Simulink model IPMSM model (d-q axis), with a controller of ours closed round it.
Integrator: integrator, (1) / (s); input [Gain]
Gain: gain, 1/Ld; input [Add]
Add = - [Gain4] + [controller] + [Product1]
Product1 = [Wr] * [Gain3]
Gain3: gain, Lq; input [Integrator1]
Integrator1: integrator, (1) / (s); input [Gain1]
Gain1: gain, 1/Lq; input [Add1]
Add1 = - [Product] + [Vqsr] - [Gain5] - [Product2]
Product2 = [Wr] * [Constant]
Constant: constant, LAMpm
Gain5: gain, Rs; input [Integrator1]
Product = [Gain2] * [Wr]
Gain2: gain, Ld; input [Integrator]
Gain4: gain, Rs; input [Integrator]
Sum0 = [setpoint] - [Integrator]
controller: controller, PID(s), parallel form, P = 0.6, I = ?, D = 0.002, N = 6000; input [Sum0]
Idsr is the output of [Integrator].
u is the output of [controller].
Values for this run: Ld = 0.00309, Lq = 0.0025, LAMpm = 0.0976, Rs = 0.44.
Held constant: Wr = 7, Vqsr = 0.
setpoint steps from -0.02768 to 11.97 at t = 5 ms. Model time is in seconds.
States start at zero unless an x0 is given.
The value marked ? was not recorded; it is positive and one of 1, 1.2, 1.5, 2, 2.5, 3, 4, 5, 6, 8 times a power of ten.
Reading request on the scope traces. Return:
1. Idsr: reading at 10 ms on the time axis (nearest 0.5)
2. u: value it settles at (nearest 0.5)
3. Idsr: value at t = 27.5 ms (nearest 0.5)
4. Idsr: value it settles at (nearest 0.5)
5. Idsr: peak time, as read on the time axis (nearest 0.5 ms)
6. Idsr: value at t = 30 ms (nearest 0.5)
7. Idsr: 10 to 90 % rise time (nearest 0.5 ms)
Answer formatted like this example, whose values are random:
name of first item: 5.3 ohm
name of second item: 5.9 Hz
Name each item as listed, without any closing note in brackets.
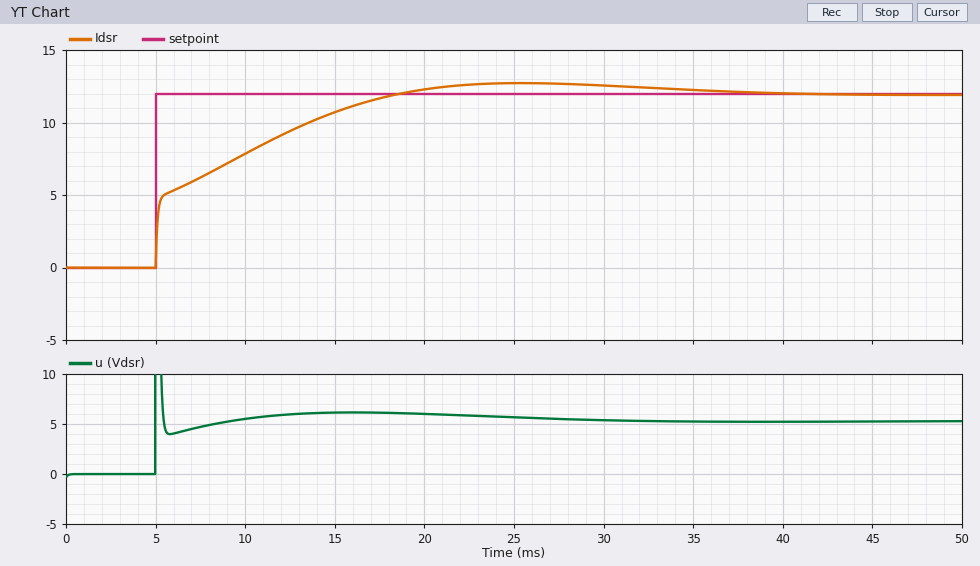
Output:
Idsr: reading at 10 ms on the time axis: 8.0
u: value it settles at: 5.5
Idsr: value at t = 27.5 ms: 12.5
Idsr: value it settles at: 12.0
Idsr: peak time, as read on the time axis: 25.5 ms
Idsr: value at t = 30 ms: 12.5
Idsr: 10 to 90 % rise time: 10.0 ms
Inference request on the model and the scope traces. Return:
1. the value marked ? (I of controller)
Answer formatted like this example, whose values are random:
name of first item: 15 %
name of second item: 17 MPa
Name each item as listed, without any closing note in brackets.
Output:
the value marked ?: 150
